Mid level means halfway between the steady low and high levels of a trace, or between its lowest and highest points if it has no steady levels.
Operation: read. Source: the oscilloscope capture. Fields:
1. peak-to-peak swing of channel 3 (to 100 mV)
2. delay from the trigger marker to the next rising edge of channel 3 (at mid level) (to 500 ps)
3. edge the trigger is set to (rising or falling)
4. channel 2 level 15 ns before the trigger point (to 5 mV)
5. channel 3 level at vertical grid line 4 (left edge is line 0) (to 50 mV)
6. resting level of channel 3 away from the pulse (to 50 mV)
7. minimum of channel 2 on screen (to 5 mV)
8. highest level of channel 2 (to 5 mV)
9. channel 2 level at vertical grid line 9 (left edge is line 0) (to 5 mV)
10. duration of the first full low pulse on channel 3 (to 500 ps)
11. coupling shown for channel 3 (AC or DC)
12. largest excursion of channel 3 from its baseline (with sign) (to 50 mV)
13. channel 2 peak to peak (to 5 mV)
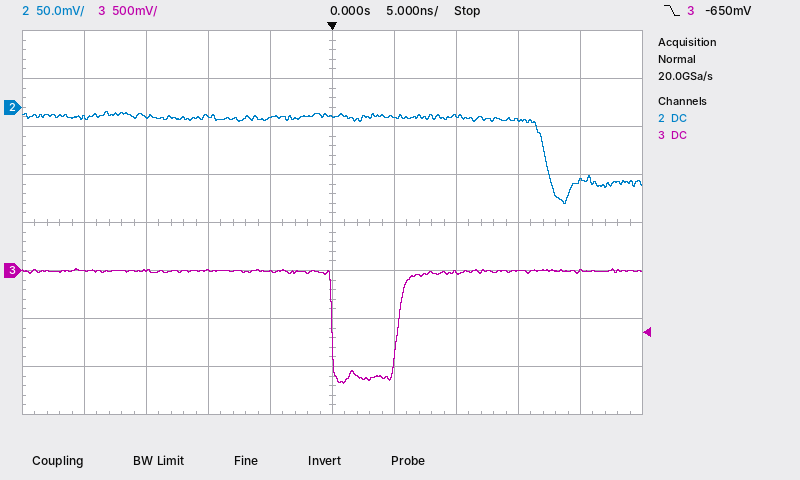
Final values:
1.20 V
5.5 ns
falling
-10 mV
0 mV
0 mV
-100 mV
-5 mV
-75 mV
5.5 ns
DC
-1.15 V
95 mV
